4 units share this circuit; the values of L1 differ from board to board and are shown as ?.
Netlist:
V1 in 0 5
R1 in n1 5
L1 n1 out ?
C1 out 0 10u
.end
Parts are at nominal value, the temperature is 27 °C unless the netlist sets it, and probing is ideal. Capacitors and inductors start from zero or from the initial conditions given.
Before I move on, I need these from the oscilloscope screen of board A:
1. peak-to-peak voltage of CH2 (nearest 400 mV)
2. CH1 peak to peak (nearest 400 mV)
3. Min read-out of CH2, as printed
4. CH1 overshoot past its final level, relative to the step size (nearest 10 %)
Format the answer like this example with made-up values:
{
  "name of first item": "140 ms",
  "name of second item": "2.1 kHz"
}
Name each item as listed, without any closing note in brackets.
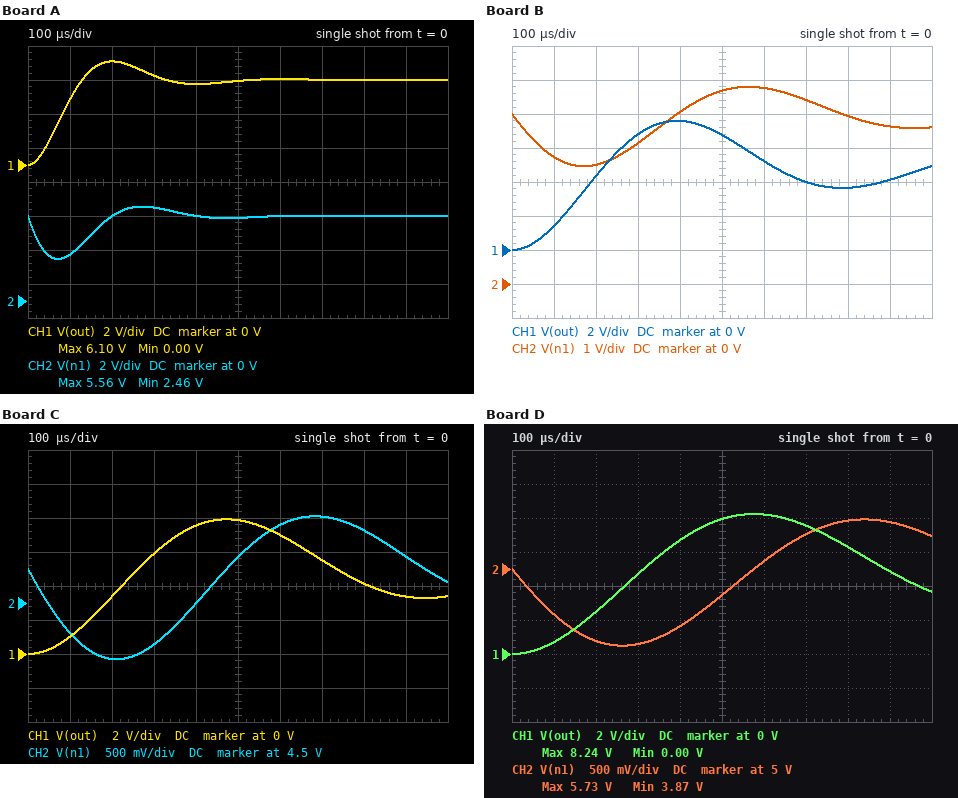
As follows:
{
  "peak-to-peak voltage of CH2": "3.2 V",
  "CH1 peak to peak": "6.0 V",
  "Min read-out of CH2, as printed": "2.46 V",
  "CH1 overshoot past its final level, relative to the step size": "20 %"
}
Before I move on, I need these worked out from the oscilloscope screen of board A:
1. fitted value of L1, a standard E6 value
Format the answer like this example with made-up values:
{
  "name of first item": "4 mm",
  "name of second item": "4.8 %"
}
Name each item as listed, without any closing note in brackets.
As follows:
{
  "fitted value of L1, a standard E6 value": "330 µH"
}
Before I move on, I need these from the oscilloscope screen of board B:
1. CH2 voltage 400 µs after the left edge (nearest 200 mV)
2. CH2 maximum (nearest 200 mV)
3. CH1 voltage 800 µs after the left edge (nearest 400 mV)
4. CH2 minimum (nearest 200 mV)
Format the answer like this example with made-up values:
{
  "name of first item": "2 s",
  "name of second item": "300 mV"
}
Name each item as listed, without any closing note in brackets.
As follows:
{
  "CH2 voltage 400 µs after the left edge": "5.0 V",
  "CH2 maximum": "5.8 V",
  "CH1 voltage 800 µs after the left edge": "3.6 V",
  "CH2 minimum": "3.4 V"
}
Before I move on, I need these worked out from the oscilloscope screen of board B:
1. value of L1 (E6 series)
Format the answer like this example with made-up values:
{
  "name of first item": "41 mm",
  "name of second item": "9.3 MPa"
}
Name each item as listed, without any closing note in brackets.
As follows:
{
  "value of L1": "1.5 mH"
}
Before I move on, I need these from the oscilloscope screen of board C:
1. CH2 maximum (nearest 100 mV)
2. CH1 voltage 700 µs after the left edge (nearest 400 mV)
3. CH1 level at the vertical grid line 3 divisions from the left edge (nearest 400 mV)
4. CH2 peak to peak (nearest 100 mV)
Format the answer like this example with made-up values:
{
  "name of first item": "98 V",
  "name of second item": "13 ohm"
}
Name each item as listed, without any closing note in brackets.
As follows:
{
  "CH2 maximum": "5.8 V",
  "CH1 voltage 700 µs after the left edge": "5.6 V",
  "CH1 level at the vertical grid line 3 divisions from the left edge": "6.0 V",
  "CH2 peak to peak": "2.1 V"
}
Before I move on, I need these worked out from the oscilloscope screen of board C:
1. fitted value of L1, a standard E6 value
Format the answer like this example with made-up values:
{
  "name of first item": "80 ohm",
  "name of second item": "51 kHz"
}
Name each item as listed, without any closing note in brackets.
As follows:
{
  "fitted value of L1, a standard E6 value": "2.2 mH"
}
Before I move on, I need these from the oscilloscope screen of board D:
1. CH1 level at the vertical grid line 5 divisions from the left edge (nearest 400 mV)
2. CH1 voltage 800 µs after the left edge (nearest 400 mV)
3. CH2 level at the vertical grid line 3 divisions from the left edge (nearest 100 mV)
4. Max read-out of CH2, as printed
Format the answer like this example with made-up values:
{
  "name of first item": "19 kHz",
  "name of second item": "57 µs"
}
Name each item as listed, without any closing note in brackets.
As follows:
{
  "CH1 level at the vertical grid line 5 divisions from the left edge": "8.0 V",
  "CH1 voltage 800 µs after the left edge": "6.4 V",
  "CH2 level at the vertical grid line 3 divisions from the left edge": "3.9 V",
  "Max read-out of CH2, as printed": "5.73 V"
}
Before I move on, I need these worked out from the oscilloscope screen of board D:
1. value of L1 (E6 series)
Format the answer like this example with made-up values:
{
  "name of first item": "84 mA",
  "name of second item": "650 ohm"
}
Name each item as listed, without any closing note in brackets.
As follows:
{
  "value of L1": "3.3 mH"
}
